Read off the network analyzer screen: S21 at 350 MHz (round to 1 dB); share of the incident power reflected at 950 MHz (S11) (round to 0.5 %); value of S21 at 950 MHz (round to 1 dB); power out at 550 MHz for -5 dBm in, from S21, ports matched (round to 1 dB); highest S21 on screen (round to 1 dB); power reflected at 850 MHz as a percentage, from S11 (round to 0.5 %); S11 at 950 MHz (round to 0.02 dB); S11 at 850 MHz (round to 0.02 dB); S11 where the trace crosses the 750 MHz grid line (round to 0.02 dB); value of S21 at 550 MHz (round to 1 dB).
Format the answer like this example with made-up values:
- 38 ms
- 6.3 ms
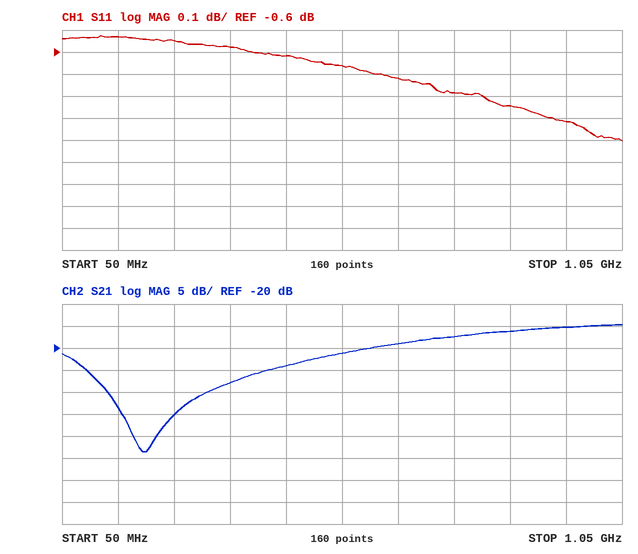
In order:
- -28 dB
- 81.0 %
- -15 dB
- -26 dBm
- -15 dB
- 82.5 %
- -0.92 dB
- -0.84 dB
- -0.78 dB
- -21 dB
